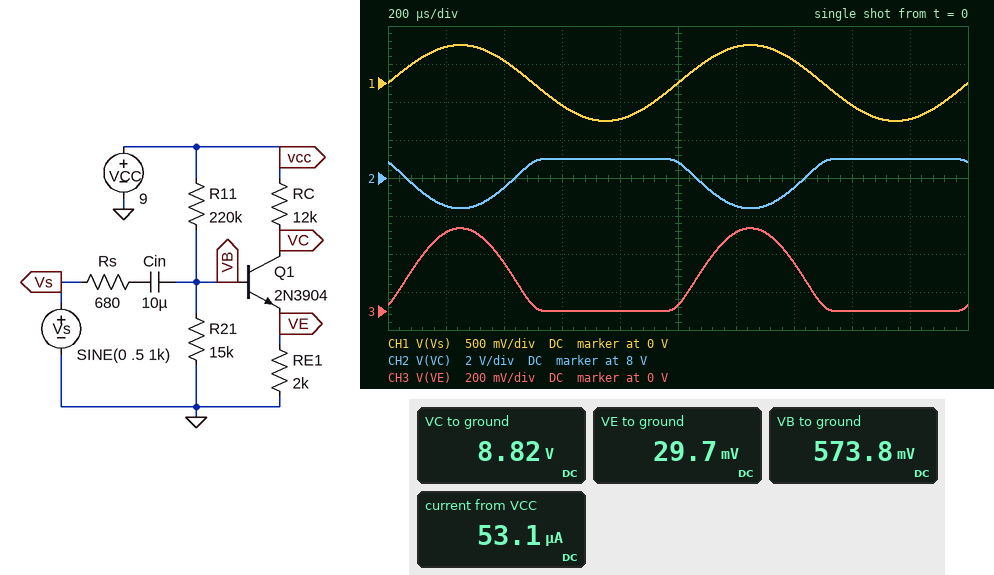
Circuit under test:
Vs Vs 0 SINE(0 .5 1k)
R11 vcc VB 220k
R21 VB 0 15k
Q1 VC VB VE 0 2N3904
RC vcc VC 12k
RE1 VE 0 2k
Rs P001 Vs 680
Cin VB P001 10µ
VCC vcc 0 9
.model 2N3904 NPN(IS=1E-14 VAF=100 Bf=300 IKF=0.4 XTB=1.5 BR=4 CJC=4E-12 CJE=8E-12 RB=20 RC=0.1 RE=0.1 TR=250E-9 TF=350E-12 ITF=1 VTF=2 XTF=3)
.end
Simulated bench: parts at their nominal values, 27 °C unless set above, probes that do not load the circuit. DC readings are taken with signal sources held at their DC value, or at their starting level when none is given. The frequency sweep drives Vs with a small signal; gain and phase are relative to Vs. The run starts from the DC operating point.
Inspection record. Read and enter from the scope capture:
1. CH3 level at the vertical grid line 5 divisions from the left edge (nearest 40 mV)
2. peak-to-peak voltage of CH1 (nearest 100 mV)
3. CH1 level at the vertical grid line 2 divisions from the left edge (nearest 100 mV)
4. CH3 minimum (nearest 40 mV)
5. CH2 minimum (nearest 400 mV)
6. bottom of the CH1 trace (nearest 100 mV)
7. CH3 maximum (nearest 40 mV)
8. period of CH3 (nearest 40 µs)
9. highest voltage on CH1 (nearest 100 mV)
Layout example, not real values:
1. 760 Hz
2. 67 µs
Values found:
1. 40 mV
2. 1.0 V
3. 300 mV
4. 0 V
5. 6.4 V
6. -500 mV
7. 440 mV
8. 1.00 ms
9. 500 mV
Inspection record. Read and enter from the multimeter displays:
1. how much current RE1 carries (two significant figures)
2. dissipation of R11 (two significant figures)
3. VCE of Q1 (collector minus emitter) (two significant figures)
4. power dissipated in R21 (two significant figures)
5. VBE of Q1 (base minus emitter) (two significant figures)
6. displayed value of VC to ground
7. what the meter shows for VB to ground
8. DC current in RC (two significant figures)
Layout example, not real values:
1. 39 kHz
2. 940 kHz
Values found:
1. 15 µA
2. 320 µW
3. 8.8 V
4. 22 µW
5. 540 mV
6. 8.82 V
7. 573.8 mV
8. 15 µA
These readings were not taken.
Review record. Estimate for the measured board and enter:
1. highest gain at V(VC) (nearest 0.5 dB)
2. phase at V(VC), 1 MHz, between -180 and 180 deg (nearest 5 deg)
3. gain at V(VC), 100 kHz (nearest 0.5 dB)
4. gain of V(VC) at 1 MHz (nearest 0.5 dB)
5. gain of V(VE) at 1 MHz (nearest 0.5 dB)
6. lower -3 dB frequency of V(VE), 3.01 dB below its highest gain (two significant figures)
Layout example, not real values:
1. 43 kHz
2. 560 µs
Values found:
1. 9.5 dB
2. 165 deg
3. 9.5 dB
4. 9.5 dB
5. -6.0 dB
6. 3.4 Hz
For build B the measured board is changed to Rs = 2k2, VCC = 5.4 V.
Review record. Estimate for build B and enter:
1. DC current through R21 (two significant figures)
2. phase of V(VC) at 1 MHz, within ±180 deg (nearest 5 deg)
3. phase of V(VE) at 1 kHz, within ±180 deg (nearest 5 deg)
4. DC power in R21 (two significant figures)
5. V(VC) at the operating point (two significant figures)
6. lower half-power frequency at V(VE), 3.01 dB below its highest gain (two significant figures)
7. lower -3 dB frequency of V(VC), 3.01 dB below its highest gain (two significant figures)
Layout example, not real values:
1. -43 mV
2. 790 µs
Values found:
1. 23 µA
2. 75 deg
3. 15 deg
4. 7.9 µW
5. 5.4 V
6. 3.9 MHz
7. 2.8 MHz
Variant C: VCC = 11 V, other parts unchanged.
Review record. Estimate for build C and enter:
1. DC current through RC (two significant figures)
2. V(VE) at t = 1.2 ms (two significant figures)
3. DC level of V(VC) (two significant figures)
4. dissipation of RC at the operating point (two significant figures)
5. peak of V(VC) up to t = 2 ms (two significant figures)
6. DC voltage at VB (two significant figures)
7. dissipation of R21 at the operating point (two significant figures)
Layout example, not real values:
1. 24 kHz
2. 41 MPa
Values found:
1. 60 µA
2. 530 mV
3. 10 V
4. 43 µW
5. 11 V
6. 700 mV
7. 33 µW
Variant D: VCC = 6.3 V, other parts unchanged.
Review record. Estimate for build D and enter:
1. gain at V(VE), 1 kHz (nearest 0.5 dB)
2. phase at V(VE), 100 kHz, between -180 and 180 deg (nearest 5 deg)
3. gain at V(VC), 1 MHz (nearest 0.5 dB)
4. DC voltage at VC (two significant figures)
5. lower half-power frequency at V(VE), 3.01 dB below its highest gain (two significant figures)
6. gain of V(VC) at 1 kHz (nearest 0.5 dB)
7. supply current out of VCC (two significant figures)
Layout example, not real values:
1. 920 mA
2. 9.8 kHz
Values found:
1. -47.0 dB
2. 70 deg
3. -17.0 dB
4. 6.3 V
5. 5.6 MHz
6. -31.5 dB
7. 27 µA
